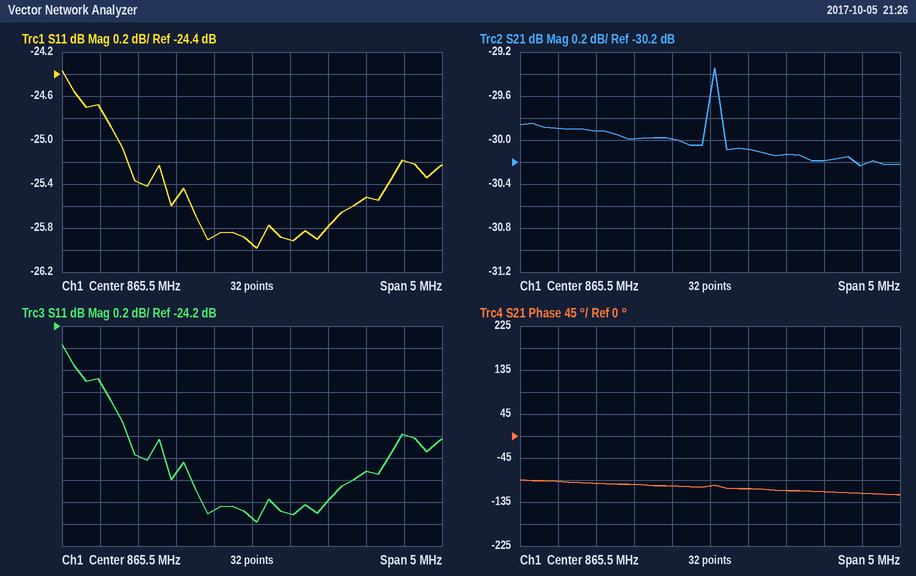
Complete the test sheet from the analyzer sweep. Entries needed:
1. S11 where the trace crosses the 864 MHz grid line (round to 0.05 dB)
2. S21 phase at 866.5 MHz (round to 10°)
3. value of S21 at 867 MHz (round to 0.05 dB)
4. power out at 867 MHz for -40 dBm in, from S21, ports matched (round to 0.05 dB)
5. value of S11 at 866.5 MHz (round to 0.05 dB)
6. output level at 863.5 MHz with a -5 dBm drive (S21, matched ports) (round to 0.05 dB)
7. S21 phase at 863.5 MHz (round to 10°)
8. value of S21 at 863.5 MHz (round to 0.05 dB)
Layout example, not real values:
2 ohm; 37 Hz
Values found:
-25.40 dB; -110°; -30.20 dB; -70.20 dBm; -25.80 dB; -34.90 dBm; -90°; -29.90 dB
